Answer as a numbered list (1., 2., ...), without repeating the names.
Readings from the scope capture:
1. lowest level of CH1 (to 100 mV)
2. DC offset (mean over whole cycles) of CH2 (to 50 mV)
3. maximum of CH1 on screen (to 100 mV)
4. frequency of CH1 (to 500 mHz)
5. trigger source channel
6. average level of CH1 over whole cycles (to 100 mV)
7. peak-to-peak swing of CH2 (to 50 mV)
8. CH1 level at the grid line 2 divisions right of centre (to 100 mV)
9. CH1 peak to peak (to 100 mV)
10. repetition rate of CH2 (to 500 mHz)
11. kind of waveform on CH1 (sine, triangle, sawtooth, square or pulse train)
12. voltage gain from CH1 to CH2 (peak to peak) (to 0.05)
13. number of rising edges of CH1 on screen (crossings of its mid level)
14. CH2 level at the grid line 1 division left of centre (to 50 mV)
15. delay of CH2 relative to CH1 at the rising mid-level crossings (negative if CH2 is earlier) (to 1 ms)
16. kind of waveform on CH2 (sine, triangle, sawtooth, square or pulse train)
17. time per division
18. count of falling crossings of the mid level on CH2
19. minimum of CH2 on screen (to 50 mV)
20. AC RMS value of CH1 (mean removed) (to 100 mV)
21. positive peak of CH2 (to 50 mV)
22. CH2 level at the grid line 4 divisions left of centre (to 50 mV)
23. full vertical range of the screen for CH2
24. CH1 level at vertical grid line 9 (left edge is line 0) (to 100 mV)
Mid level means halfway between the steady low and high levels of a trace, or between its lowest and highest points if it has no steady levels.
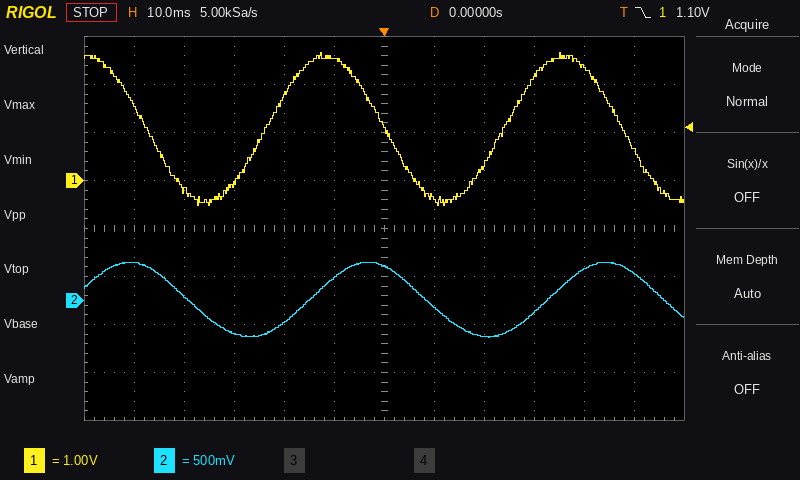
1. -500 mV
2. 0 mV
3. 2.7 V
4. 21.0 Hz
5. CH1
6. 1.1 V
7. 800 mV
8. 300 mV
9. 3.2 V
10. 21.0 Hz
11. sine
12. 0.25
13. 2
14. 250 mV
15. +9 ms
16. sine
17. 10 ms
18. 3
19. -400 mV
20. 1.1 V
21. 400 mV
22. 50 mV
23. 4 V
24. 2.2 V
